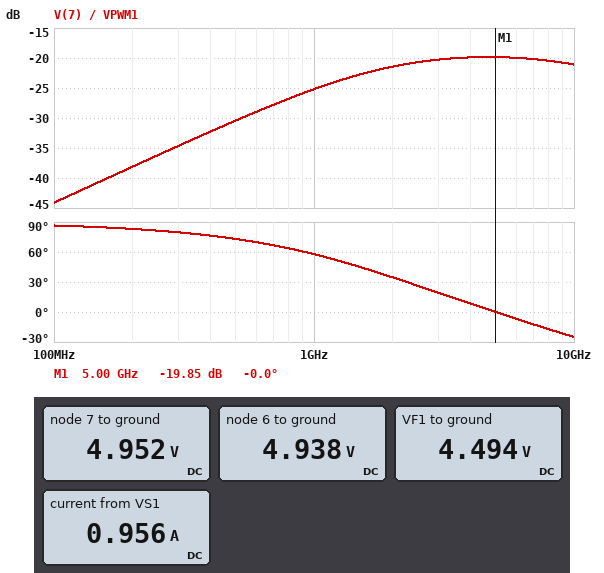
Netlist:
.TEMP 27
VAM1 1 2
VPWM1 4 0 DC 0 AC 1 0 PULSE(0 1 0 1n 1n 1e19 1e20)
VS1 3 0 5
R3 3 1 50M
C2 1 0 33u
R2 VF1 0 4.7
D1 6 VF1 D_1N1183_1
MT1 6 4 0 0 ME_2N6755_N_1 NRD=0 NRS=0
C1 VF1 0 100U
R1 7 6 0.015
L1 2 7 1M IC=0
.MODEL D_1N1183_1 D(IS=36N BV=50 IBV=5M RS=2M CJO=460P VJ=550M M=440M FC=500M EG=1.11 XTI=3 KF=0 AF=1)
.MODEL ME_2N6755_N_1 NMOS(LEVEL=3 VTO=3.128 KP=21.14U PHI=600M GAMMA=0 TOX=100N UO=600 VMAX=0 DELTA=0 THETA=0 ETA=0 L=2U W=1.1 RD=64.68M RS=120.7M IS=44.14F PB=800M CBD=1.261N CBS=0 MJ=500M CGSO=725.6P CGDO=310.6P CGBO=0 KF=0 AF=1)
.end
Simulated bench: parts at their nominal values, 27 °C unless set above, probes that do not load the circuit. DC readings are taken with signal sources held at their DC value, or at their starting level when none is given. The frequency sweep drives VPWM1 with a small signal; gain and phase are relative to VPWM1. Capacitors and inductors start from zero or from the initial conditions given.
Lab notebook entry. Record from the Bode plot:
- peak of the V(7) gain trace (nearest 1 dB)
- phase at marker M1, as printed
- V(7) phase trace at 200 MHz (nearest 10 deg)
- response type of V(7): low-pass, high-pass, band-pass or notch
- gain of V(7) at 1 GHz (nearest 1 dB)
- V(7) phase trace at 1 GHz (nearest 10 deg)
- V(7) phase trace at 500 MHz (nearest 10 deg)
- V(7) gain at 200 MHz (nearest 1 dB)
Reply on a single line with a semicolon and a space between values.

-20 dB; -0.0 deg; 80 deg; high-pass; -25 dB; 60 deg; 70 deg; -38 dB
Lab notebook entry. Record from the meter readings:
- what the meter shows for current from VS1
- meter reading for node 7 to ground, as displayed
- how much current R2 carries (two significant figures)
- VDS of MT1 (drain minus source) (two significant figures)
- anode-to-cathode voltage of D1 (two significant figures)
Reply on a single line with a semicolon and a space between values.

0.956 A; 4.952 V; 960 mA; 4.9 V; 440 mV
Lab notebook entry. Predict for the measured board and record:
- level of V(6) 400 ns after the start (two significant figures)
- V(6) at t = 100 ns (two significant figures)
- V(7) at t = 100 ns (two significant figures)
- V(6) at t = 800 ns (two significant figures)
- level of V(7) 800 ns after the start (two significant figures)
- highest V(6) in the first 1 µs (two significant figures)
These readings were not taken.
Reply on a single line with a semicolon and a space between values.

170 mV; 170 mV; 170 mV; 230 mV; 230 mV; 260 mV
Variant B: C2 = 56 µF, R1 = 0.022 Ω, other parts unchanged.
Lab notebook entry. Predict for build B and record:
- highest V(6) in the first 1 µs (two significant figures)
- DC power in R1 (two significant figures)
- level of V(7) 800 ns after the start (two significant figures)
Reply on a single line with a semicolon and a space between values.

230 mV; 20 mW; 200 mV
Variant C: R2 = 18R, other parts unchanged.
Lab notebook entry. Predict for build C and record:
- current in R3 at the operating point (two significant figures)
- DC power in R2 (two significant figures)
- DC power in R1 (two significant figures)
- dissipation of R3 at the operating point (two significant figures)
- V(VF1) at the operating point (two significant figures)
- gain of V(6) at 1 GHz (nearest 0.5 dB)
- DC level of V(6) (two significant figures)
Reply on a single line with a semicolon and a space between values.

250 mA; 1.2 W; 970 µW; 3.2 mW; 4.6 V; -17.0 dB; 5.0 V
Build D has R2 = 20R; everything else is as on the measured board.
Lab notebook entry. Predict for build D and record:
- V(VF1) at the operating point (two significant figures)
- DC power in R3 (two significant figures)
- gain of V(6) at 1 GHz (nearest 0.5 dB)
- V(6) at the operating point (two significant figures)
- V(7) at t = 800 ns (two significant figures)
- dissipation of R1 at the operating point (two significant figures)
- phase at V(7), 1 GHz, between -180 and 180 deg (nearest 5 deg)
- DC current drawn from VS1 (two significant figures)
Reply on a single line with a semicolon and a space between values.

4.6 V; 2.6 mW; -16.5 dB; 5.0 V; 230 mV; 790 µW; 30 deg; 230 mA
